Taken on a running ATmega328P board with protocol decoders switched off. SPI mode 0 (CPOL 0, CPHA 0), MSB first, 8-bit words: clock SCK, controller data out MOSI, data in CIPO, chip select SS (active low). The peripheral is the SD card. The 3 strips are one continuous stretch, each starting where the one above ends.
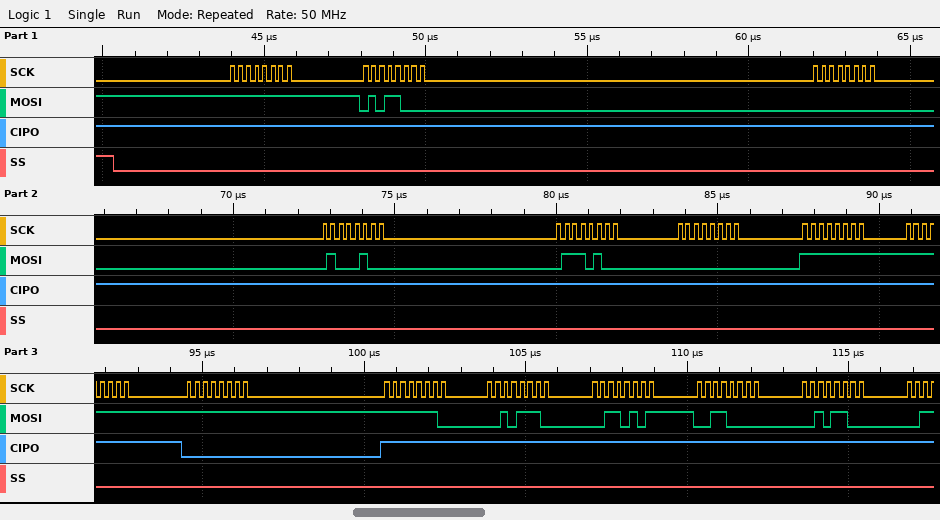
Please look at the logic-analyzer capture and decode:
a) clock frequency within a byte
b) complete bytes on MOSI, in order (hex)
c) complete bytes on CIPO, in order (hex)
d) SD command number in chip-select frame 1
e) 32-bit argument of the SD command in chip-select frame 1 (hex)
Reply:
4 MHz
FF 58 00 44 74 00 FF FF FF FE 2E 35 30 2C
FF FF FF FF FF FF FF FF 00 FF FF FF FF FF
CMD24
0x00447400
